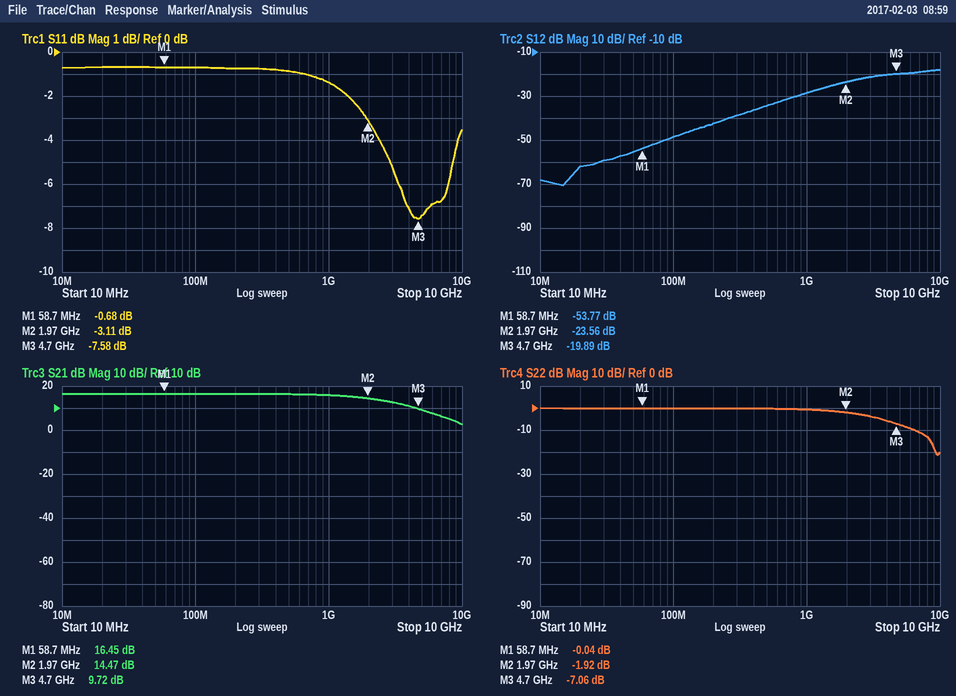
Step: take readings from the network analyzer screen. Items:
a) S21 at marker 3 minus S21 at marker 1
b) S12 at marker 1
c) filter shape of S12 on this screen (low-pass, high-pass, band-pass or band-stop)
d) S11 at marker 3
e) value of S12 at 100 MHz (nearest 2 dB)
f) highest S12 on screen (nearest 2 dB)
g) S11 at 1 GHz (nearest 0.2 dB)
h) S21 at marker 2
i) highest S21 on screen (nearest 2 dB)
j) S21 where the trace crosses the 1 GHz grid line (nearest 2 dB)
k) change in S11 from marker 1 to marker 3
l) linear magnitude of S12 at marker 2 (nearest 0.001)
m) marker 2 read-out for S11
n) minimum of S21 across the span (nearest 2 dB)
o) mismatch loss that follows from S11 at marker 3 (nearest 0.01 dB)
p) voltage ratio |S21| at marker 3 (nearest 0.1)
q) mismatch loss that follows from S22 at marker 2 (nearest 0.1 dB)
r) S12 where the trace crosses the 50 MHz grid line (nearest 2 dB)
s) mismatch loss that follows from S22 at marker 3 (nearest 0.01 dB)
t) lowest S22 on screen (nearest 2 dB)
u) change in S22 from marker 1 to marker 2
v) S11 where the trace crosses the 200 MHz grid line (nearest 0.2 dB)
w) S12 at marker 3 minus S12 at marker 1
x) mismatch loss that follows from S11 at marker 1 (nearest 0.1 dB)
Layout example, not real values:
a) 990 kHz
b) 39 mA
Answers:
a) -6.73 dB
b) -53.77 dB
c) high-pass
d) -7.58 dB
e) -48 dB
f) -18 dB
g) -1.4 dB
h) 14.47 dB
i) 16 dB
j) 16 dB
k) -6.90 dB
l) 0.066
m) -3.11 dB
n) 2 dB
o) 0.83 dB
p) 3.1
q) 4.5 dB
r) -56 dB
s) 0.95 dB
t) -22 dB
u) -1.88 dB
v) -0.8 dB
w) 33.88 dB
x) 8.4 dB
